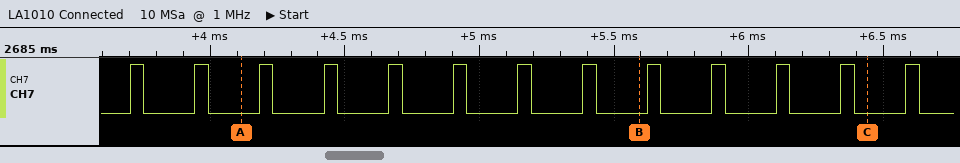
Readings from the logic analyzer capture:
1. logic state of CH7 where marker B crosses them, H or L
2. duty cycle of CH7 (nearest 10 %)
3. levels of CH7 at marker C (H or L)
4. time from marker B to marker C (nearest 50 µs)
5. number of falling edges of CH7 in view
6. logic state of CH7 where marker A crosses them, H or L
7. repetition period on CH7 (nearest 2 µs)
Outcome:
CH7=L
20 %
CH7=L
850 µs
13
CH7=L
240 µs
